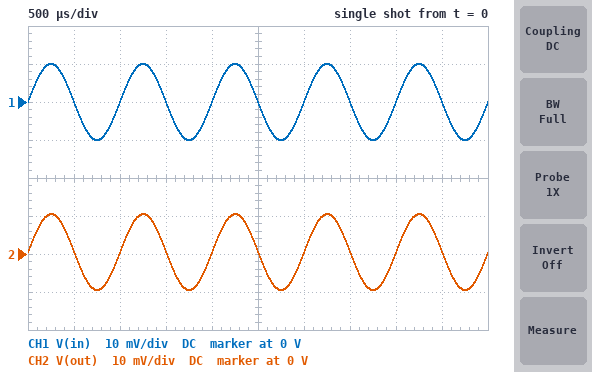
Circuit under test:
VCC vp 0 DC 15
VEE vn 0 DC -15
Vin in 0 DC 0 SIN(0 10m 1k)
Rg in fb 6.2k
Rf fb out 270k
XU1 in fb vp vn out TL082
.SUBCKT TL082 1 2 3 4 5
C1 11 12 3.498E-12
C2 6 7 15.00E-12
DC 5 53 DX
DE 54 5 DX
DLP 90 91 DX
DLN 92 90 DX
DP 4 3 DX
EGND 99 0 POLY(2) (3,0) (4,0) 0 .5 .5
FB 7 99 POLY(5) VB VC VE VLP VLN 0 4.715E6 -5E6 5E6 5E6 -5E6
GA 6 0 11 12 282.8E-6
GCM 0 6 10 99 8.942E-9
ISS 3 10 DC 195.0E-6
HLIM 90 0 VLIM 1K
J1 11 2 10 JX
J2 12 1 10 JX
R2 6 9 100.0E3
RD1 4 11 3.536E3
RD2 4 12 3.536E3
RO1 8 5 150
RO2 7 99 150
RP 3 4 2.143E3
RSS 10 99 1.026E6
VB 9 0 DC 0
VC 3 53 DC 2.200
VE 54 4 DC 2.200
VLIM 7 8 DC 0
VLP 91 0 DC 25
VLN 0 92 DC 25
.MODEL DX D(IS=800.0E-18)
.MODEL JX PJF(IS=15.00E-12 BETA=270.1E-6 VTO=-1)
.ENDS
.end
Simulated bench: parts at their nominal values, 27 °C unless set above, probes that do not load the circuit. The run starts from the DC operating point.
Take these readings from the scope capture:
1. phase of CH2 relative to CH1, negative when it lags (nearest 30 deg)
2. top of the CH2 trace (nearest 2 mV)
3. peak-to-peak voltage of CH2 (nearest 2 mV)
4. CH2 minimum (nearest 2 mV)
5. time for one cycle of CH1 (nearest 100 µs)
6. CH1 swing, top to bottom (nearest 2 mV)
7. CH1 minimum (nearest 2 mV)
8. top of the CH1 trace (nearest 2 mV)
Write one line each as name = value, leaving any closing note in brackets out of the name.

phase of CH2 relative to CH1, negative when it lags = 0 deg
top of the CH2 trace = 10 mV
peak-to-peak voltage of CH2 = 20 mV
CH2 minimum = -10 mV
time for one cycle of CH1 = 1.0 ms
CH1 swing, top to bottom = 20 mV
CH1 minimum = -10 mV
top of the CH1 trace = 10 mV
